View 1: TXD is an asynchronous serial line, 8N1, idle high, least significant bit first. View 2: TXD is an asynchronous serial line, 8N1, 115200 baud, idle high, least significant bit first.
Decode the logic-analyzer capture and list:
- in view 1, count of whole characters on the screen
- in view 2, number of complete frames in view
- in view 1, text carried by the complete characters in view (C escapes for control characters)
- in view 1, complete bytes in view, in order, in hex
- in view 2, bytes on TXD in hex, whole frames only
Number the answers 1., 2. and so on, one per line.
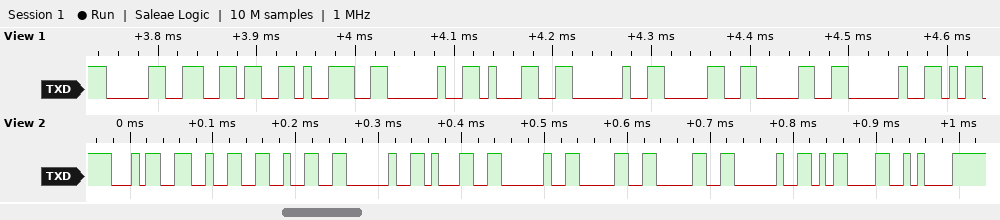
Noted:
1. 9
2. 11
3. "069 1 00 "
4. 0x30 0x36 0x39 0x20 0x31 0x20 0x30 0x30 0x20
5. 34 32 32 20 31 20 30 30 20 0D 0A
